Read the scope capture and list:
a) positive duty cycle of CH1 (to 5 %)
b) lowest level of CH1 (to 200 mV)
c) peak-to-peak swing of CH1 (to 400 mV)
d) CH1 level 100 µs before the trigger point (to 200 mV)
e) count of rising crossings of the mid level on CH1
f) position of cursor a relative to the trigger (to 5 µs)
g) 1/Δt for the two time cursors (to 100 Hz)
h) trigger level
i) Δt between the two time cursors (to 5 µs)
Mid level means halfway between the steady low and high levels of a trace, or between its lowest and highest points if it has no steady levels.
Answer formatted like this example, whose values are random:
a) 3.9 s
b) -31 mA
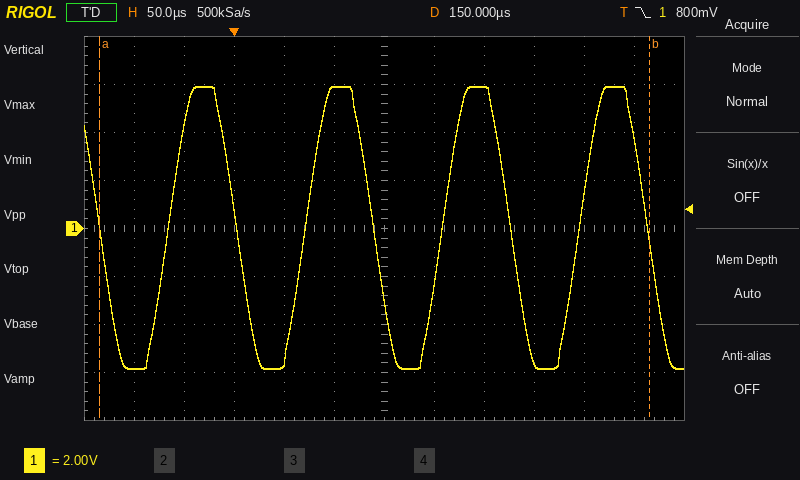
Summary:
a) 50 %
b) -5.8 V
c) 11.6 V
d) -5.8 V
e) 4
f) -135 µs
g) 1.8 kHz
h) 800 mV
i) 550 µs
